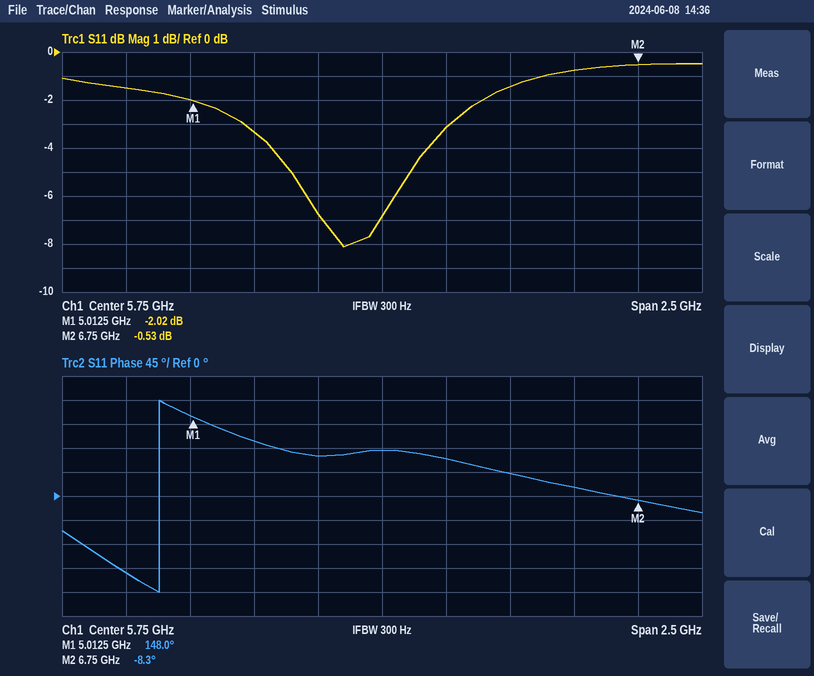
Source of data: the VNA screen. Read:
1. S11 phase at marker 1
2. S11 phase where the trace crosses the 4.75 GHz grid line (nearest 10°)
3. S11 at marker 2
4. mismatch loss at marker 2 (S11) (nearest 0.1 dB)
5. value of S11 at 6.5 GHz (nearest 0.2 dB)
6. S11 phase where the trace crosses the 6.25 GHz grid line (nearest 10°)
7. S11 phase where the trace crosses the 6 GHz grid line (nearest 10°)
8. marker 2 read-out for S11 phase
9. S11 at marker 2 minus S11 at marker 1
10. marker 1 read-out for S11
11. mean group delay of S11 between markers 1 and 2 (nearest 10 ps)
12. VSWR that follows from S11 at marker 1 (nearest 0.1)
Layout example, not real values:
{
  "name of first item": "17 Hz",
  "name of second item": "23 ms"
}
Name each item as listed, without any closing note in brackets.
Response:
{
  "S11 phase at marker 1": "148.0°",
  "S11 phase where the trace crosses the 4.75 GHz grid line": "-140°",
  "S11 at marker 2": "-0.53 dB",
  "mismatch loss at marker 2 (S11)": "9.4 dB",
  "value of S11 at 6.5 GHz": "-0.8 dB",
  "S11 phase where the trace crosses the 6.25 GHz grid line": "40°",
  "S11 phase where the trace crosses the 6 GHz grid line": "70°",
  "marker 2 read-out for S11 phase": "-8.3°",
  "S11 at marker 2 minus S11 at marker 1": "1.49 dB",
  "marker 1 read-out for S11": "-2.02 dB",
  "mean group delay of S11 between markers 1 and 2": "250 ps",
  "VSWR that follows from S11 at marker 1": "8.6"
}
